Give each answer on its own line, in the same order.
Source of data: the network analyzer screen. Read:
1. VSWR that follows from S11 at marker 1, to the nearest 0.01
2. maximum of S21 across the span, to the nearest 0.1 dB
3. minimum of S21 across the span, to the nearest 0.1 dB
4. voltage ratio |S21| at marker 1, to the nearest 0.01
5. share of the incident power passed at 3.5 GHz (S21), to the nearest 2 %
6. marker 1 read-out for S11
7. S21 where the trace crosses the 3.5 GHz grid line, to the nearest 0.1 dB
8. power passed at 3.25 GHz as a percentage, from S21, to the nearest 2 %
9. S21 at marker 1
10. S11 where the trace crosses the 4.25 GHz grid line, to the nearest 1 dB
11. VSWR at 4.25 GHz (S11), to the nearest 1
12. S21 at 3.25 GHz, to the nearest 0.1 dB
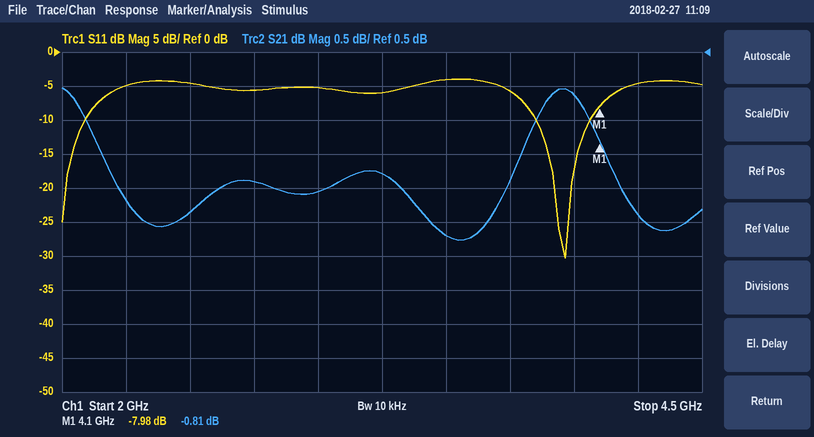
2.33
0.0 dB
-2.3 dB
0.91
60 %
-7.98 dB
-2.2 dB
74 %
-0.81 dB
-5 dB
4
-1.3 dB
